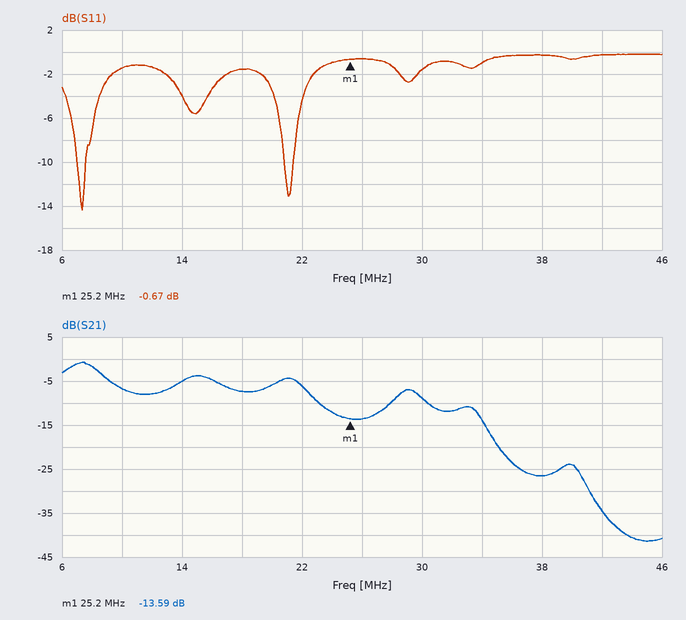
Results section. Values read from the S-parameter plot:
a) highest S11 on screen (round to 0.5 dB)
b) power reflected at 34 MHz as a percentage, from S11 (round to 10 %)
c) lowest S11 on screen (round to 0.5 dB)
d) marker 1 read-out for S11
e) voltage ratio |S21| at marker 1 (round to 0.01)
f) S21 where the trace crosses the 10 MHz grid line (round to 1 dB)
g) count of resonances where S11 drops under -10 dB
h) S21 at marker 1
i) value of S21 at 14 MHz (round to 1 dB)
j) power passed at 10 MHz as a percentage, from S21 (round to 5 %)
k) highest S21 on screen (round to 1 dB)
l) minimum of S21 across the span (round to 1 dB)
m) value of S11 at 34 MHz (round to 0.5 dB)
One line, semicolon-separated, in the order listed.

0.0 dB; 80 %; -14.5 dB; -0.67 dB; 0.21; -7 dB; 2; -13.59 dB; -5 dB; 20 %; -1 dB; -41 dB; -1.0 dB
